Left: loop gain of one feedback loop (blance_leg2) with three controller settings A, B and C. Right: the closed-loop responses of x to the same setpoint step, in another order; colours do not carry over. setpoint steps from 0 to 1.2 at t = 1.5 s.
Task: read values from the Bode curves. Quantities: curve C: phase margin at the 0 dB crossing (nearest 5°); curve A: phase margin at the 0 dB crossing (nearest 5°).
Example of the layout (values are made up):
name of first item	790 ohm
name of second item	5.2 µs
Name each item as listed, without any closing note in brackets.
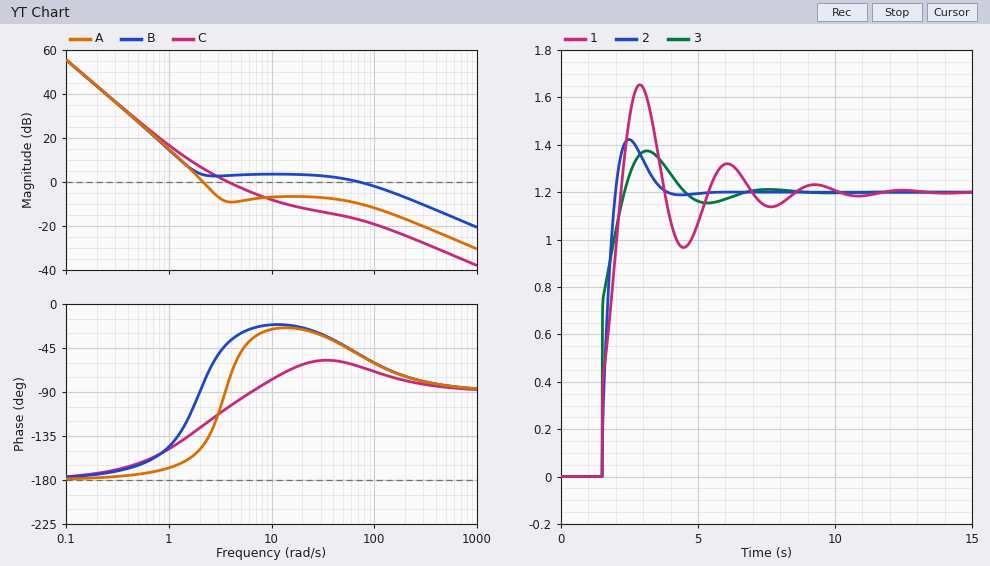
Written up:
curve C: phase margin at the 0 dB crossing	75°
curve A: phase margin at the 0 dB crossing	35°
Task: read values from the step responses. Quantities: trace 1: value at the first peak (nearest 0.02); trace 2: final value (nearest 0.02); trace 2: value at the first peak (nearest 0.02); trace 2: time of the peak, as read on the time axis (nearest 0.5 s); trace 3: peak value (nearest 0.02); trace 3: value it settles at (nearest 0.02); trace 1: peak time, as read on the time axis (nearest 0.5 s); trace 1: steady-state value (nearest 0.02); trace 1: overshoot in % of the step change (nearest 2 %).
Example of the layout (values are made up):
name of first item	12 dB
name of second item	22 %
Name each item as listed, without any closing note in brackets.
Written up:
trace 1: value at the first peak	1.66
trace 2: final value	1.20
trace 2: value at the first peak	1.42
trace 2: time of the peak, as read on the time axis	2.5 s
trace 3: peak value	1.38
trace 3: value it settles at	1.20
trace 1: peak time, as read on the time axis	3.0 s
trace 1: steady-state value	1.20
trace 1: overshoot in % of the step change	38 %
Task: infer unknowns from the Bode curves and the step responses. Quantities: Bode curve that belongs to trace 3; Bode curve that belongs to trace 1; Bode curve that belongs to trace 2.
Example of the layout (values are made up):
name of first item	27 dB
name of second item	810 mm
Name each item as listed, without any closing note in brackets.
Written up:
Bode curve that belongs to trace 3	B
Bode curve that belongs to trace 1	A
Bode curve that belongs to trace 2	C
